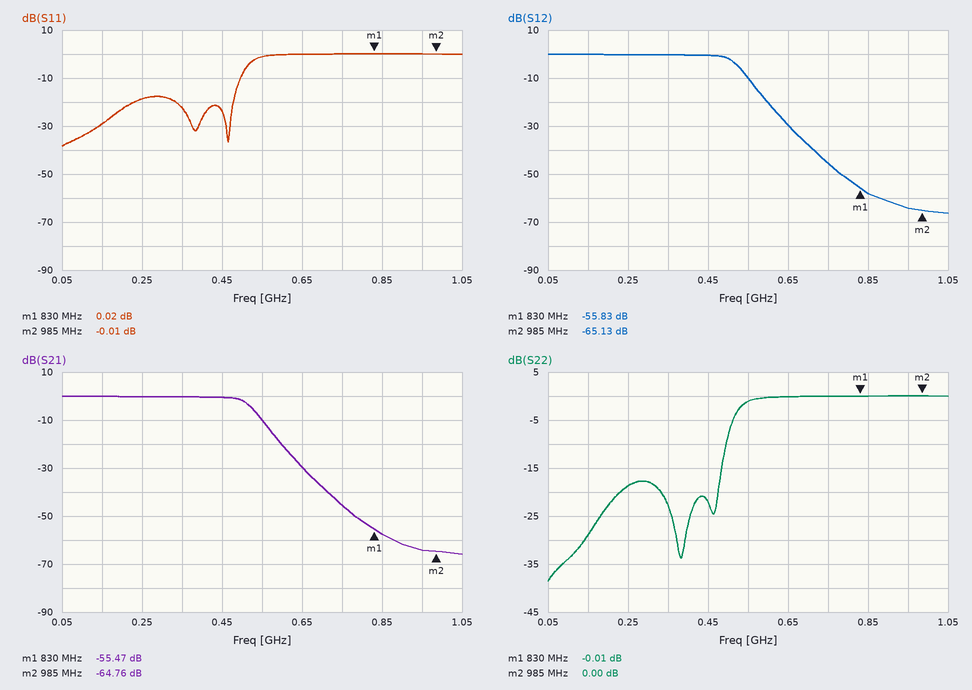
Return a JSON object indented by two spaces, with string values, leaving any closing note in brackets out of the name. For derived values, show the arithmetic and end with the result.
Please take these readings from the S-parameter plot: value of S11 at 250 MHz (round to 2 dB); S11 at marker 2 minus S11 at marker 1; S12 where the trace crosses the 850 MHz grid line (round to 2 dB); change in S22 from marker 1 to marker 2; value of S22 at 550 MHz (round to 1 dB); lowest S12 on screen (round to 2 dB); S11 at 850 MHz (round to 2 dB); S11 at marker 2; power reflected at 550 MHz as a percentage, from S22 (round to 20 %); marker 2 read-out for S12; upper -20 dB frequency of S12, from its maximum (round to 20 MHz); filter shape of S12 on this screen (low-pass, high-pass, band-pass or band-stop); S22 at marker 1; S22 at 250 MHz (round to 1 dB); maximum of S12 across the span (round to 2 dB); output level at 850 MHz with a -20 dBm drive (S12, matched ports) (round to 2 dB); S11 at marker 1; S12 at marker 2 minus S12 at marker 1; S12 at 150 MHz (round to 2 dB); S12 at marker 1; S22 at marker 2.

{
  "value of S11 at 250 MHz": "-18 dB",
  "S11 at marker 2 minus S11 at marker 1": "-0.01 − (0.02) = -0.03 dB",
  "S12 where the trace crosses the 850 MHz grid line": "-58 dB",
  "change in S22 from marker 1 to marker 2": "0 − (-0.01) = 0.01 dB",
  "value of S22 at 550 MHz": "-1 dB",
  "lowest S12 on screen": "-66 dB",
  "S11 at 850 MHz": "0 dB",
  "S11 at marker 2": "-0.01 dB",
  "power reflected at 550 MHz as a percentage, from S22": "10^(-1/10) ≈ 79.4 %, so 80 % to the nearest 20 %",
  "marker 2 read-out for S12": "-65.13 dB",
  "upper -20 dB frequency of S12, from its maximum": "600 MHz",
  "filter shape of S12 on this screen": "low-pass",
  "S22 at marker 1": "-0.01 dB",
  "S22 at 250 MHz": "-19 dB",
  "maximum of S12 across the span": "0 dB",
  "output level at 850 MHz with a -20 dBm drive (S12, matched ports)": "-20 dBm + (-58 dB) = -78 dBm",
  "S11 at marker 1": "0.02 dB",
  "S12 at marker 2 minus S12 at marker 1": "-65.13 − (-55.83) = -9.30 dB",
  "S12 at 150 MHz": "0 dB",
  "S12 at marker 1": "-55.83 dB",
  "S22 at marker 2": "0.00 dB"
}
